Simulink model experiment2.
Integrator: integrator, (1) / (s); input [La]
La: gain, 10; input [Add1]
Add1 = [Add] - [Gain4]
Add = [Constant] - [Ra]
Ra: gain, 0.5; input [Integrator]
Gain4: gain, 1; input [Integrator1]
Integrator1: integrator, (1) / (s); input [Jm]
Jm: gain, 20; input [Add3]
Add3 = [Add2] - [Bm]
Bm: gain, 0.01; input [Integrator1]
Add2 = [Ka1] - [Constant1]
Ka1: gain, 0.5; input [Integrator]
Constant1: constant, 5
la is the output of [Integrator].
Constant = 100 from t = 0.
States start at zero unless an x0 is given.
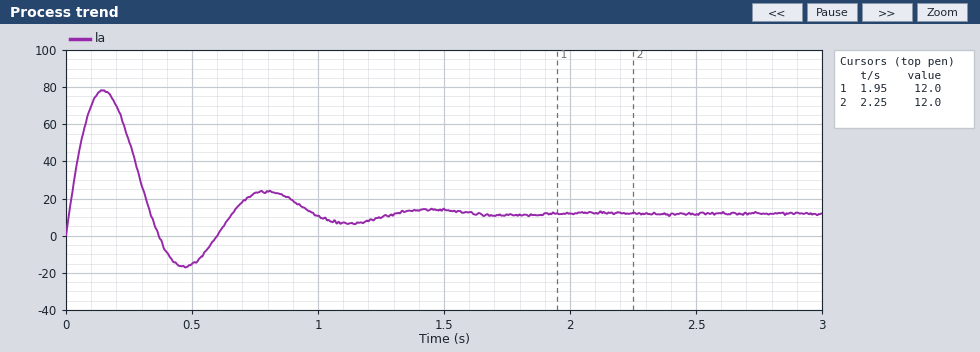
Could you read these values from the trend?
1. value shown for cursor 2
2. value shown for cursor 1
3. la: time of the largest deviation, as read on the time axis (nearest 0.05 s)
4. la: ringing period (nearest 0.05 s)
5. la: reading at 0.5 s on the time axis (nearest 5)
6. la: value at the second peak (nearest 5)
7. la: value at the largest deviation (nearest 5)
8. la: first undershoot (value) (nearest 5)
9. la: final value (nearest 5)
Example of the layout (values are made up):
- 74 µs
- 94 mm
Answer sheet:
- 12.0
- 12.0
- 0.15 s
- 0.65 s
- -15
- 25
- 80
- -15
- 10
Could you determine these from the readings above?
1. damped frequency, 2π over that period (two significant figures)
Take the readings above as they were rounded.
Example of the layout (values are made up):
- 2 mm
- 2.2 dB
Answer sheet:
- 9.7 rad/s
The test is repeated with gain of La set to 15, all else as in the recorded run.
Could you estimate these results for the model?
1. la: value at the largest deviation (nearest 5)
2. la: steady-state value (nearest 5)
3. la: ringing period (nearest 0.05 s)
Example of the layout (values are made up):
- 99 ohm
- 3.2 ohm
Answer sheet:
- 90
- 10
- 0.55 s
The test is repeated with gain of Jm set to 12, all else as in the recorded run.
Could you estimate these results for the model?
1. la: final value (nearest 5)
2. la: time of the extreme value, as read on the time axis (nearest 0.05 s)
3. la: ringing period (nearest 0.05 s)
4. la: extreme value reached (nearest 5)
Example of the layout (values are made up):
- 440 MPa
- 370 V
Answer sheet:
- 10
- 0.20 s
- 0.85 s
- 90
